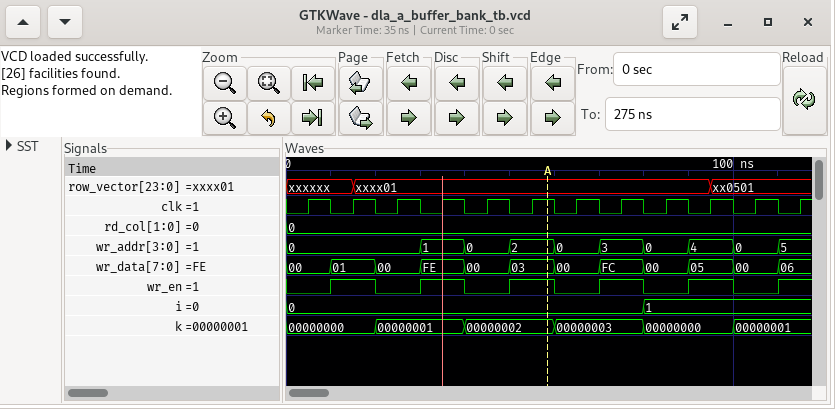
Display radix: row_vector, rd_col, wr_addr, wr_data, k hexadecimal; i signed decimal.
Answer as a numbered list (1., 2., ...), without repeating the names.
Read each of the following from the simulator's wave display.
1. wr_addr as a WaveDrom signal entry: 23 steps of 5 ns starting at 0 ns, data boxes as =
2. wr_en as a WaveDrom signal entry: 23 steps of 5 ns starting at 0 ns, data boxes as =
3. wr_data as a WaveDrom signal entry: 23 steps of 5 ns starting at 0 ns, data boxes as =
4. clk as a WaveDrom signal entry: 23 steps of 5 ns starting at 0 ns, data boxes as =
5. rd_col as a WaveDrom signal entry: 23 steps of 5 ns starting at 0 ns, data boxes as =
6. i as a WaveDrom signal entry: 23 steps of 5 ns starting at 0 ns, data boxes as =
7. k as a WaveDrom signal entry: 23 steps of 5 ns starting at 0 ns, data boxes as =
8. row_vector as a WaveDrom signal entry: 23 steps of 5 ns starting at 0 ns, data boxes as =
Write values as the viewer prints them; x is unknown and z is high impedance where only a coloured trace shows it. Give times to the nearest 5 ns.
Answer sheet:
1. {name: 'wr_addr', wave: '=.....=.=.=.=.=.=.=.=.=', data: '0 1 0 2 0 3 0 4 0 5'}
2. {name: 'wr_en', wave: '0.1.0.1.0.1.0.1.0.1.0.1'}
3. {name: 'wr_data', wave: '=.=.=.=.=.=.=.=.=.=.=.=', data: '00 01 00 FE 00 03 00 FC 00 05 00 06'}
4. {name: 'clk', wave: '01010101010101010101010'}
5. {name: 'rd_col', wave: '=......................', data: '0'}
6. {name: 'i', wave: '=...............=......', data: '0 1'}
7. {name: 'k', wave: '=...=...=...=...=...=..', data: '00000000 00000001 00000002 00000003 00000000 00000001'}
8. {name: 'row_vector', wave: 'x..=...............=...', data: 'xxxx01 xx0501'}
